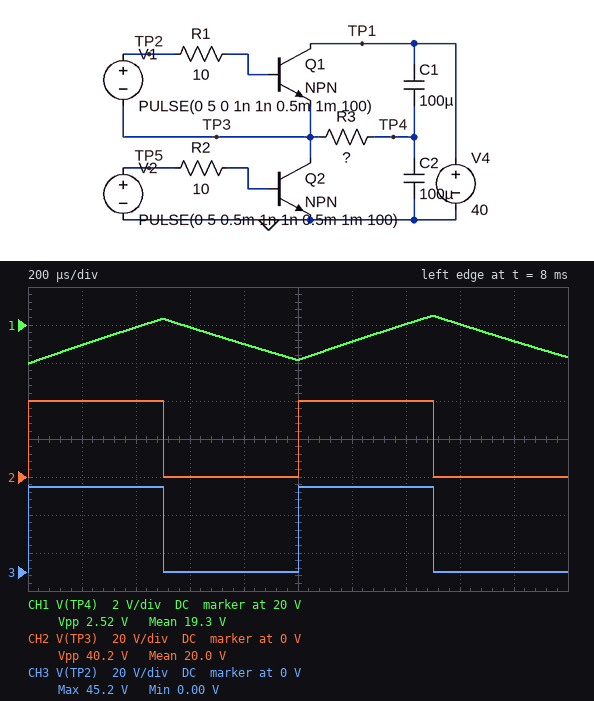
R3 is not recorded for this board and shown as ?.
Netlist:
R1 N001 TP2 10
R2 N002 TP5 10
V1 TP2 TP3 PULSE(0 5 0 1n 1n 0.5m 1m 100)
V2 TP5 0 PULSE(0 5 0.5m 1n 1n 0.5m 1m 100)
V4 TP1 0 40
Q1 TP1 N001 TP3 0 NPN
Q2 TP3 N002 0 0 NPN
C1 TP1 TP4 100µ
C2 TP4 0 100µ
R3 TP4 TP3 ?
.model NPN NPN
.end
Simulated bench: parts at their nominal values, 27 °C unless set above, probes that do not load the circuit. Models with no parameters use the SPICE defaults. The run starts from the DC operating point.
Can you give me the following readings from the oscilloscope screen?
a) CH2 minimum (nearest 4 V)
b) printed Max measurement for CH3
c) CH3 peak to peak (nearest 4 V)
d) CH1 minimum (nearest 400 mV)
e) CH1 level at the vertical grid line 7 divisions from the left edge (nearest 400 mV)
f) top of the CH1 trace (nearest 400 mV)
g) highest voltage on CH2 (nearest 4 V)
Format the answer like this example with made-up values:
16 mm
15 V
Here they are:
0 V
45.2 V
44 V
18.0 V
20.0 V
20.4 V
40 V
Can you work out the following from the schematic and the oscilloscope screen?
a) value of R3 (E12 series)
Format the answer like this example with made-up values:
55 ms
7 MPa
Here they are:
22 Ω
